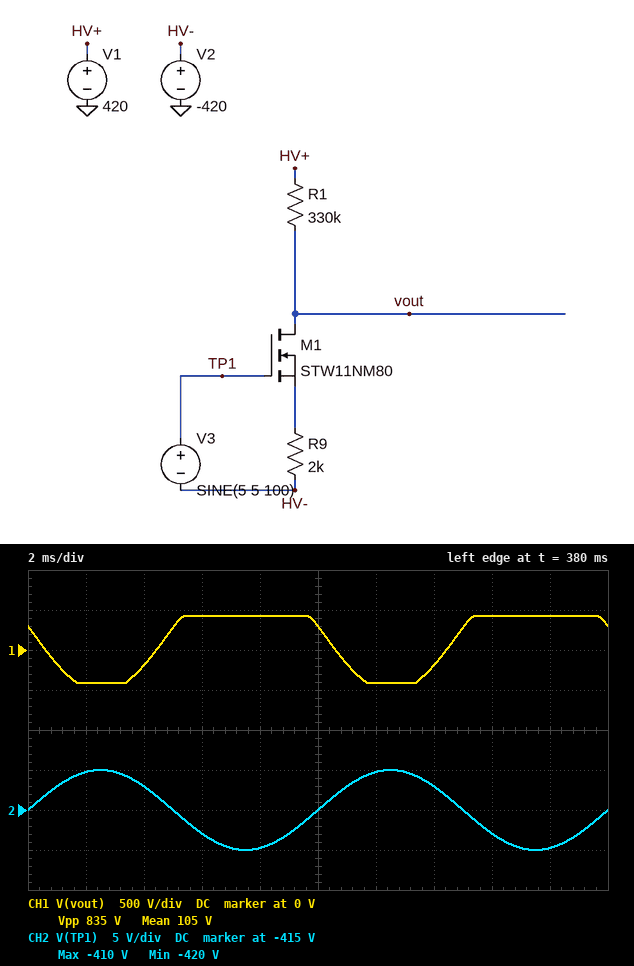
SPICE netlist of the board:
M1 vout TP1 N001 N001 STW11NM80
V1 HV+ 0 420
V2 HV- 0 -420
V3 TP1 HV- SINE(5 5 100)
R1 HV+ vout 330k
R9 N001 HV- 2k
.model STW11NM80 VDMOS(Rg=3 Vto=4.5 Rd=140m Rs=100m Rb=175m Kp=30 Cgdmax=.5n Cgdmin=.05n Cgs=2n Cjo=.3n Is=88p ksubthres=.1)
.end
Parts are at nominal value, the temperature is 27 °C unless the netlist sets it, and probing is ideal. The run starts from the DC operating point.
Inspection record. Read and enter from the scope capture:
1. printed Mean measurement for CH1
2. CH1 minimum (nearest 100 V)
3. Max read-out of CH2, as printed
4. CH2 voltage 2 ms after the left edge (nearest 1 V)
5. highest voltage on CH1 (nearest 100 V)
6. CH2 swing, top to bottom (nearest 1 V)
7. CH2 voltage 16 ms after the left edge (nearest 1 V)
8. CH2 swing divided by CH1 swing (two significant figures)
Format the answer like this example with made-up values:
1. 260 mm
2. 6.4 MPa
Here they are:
1. 105 V
2. -400 V
3. -410 V
4. -410 V
5. 400 V
6. 10 V
7. -418 V
8. 0.012
